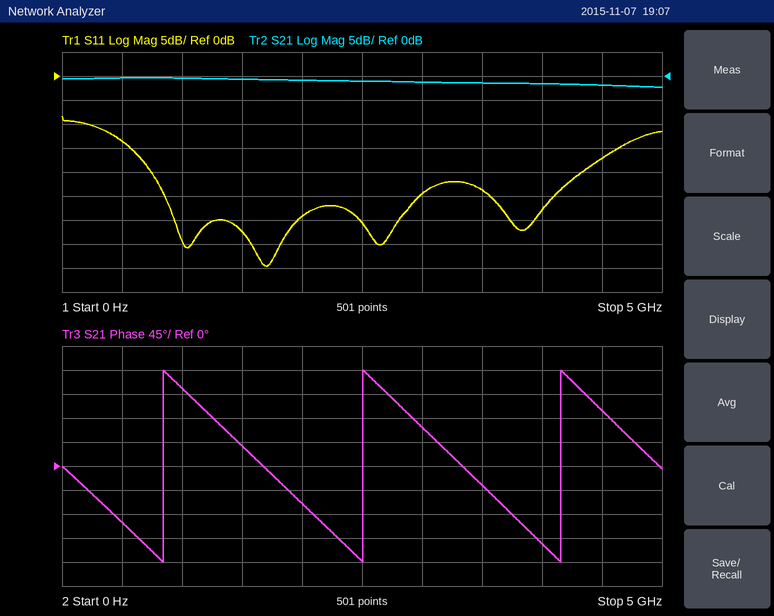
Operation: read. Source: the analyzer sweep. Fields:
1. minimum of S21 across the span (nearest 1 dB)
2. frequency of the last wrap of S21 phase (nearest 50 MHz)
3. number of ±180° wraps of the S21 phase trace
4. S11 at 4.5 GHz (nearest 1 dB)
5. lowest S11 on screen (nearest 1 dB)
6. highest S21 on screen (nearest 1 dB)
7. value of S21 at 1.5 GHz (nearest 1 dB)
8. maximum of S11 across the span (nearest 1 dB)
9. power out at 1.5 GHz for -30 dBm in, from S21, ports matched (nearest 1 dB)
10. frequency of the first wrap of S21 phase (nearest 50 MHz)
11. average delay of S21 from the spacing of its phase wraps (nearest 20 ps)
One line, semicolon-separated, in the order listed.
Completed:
-2 dB; 4.15 GHz; 3; -17 dB; -40 dB; 0 dB; -1 dB; -8 dB; -31 dBm; 850 MHz; 600 ps
